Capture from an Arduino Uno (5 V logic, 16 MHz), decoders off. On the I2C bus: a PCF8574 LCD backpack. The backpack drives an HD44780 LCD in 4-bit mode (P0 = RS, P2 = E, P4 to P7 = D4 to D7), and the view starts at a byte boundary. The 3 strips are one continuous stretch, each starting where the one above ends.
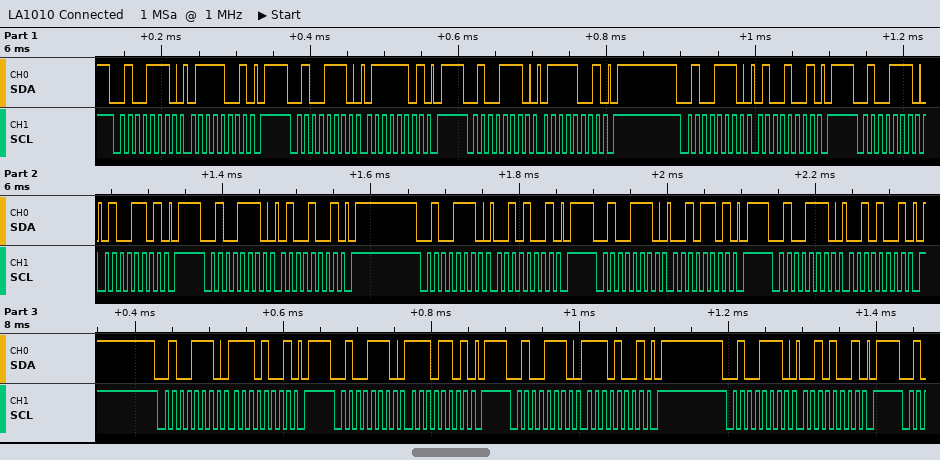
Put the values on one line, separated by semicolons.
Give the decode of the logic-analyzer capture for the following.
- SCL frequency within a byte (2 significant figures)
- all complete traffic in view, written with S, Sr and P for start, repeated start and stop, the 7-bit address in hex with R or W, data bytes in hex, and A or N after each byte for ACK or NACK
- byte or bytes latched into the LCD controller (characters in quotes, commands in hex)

100 kHz; S 27W A 79 A P S 27W A 7D A P S 27W A 79 A P S 27W A 49 A P S 27W A 4D A P S 27W A 49 A P S 27W A 29 A P S 27W A 2D A P S 27W A 29 A P S 27W A E9 A P S 27W A ED A P S 27W A E9 A P S 27W A 29 A P; 't' '.'
